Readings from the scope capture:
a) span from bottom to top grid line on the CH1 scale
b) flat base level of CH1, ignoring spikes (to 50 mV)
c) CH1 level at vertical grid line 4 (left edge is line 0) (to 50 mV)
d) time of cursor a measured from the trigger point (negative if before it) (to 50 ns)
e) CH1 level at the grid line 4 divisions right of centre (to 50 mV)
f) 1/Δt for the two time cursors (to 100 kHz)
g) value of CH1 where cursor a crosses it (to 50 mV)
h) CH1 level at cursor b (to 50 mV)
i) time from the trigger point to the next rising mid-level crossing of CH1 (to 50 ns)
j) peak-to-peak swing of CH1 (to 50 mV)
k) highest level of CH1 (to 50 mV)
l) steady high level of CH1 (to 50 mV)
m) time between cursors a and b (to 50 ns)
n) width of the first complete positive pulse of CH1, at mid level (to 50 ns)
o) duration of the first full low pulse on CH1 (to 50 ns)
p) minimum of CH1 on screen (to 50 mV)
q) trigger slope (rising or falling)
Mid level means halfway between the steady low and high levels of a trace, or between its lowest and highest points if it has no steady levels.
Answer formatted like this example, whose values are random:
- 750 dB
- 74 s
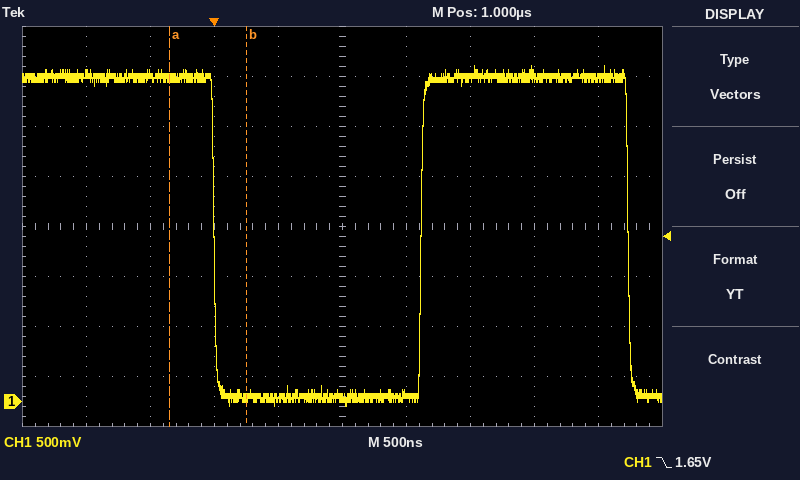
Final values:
- 4 V
- 50 mV
- 50 mV
- -350 ns
- 3.25 V
- 1.7 MHz
- 3.25 V
- 50 mV
- 1.60 µs
- 3.40 V
- 3.35 V
- 3.25 V
- 600 ns
- 1.60 µs
- 1.60 µs
- -50 mV
- falling
